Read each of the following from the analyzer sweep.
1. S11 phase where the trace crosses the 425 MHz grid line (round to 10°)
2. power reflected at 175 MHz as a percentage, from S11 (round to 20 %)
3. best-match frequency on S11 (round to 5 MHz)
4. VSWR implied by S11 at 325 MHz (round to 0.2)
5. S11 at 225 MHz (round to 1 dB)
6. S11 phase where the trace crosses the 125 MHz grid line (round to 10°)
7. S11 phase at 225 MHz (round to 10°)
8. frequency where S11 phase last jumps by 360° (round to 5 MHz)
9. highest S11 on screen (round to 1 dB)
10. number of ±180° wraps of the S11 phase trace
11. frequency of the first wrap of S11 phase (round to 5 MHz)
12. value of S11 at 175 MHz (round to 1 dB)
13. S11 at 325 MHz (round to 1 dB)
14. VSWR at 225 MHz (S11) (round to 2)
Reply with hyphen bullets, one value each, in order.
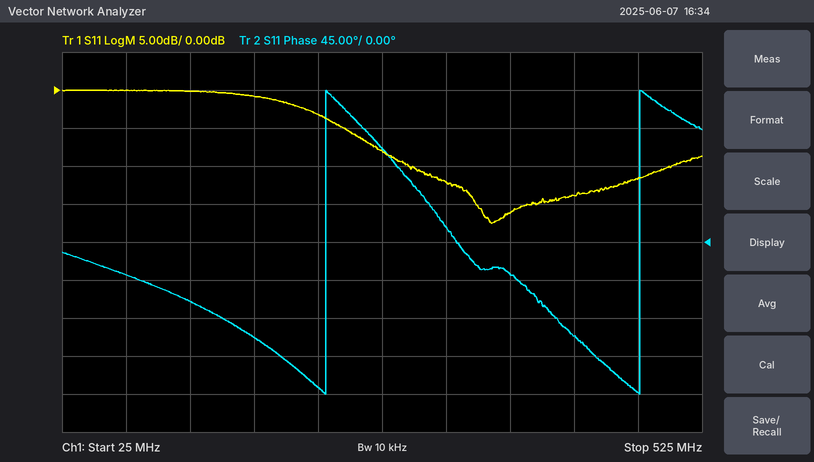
- -110°
- 80 %
- 360 MHz
- 1.6
- -3 dB
- -70°
- -170°
- 475 MHz
- 0 dB
- 2
- 230 MHz
- -1 dB
- -12 dB
- 6
